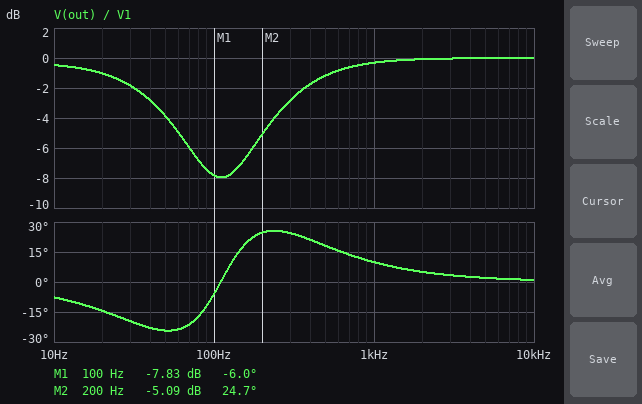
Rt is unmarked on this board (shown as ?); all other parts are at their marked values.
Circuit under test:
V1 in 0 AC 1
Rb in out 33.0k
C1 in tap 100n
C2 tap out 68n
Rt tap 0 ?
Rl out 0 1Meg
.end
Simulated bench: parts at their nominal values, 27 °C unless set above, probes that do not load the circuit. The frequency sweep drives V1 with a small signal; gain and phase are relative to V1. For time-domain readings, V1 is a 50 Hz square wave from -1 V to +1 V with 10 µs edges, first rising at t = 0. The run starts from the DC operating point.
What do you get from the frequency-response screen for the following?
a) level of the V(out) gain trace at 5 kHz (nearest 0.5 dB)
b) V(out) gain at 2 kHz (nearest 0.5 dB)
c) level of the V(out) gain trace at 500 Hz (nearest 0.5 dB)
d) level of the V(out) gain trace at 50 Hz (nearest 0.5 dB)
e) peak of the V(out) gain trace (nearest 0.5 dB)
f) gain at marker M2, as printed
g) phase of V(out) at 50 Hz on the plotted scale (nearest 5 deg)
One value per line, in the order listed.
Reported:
0 dB
0 dB
-1.0 dB
-4.0 dB
0 dB
-5.09 dB
-25 deg
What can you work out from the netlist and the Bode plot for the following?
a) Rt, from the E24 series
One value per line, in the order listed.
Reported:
9.1 kΩ
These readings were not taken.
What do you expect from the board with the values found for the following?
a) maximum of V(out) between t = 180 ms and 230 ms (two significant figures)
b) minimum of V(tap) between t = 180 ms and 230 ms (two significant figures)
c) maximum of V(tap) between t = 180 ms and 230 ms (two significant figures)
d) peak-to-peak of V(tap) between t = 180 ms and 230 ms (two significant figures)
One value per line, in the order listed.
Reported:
1.1 V
-2.0 V
2.0 V
3.9 V
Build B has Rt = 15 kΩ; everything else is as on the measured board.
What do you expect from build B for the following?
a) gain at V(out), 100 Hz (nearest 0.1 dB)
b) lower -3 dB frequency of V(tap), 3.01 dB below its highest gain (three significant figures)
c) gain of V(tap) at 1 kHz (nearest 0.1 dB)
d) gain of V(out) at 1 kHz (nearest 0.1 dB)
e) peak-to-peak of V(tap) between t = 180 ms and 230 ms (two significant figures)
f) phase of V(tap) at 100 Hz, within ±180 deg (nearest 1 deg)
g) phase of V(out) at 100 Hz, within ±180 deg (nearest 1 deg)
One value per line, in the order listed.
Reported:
-5.5 dB
111 Hz
-0.1 dB
-0.2 dB
3.8 V
34 deg
6 deg
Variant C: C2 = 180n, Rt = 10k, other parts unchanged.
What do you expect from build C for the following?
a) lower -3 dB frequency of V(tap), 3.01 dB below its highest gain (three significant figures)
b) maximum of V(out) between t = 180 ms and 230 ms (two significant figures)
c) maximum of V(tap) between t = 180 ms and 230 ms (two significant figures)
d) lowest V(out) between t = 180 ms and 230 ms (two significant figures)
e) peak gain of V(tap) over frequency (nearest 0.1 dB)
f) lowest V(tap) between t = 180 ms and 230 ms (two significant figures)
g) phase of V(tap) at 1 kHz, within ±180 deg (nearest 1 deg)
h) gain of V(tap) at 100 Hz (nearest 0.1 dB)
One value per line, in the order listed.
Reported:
190 Hz
1.4 V
1.9 V
-1.4 V
0 dB
-1.9 V
9 deg
-5.7 dB
